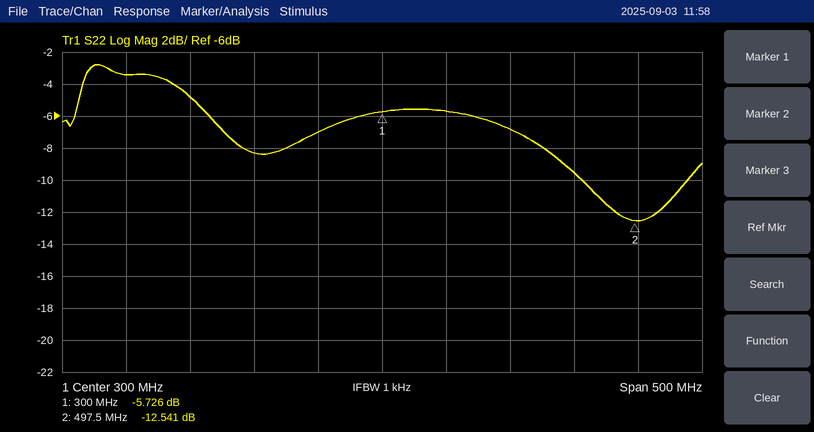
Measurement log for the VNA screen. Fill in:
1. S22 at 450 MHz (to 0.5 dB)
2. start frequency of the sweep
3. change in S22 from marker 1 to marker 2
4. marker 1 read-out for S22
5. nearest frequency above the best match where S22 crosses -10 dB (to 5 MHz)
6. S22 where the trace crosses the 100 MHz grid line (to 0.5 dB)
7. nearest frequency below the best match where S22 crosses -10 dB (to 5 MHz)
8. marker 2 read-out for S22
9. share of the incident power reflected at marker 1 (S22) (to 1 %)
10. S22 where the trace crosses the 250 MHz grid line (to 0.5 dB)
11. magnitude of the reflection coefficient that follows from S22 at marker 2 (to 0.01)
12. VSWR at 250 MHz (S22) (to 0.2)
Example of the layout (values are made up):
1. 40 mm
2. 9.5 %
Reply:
1. -9.5 dB
2. 50 MHz
3. -6.815 dB
4. -5.726 dB
5. 540 MHz
6. -3.5 dB
7. 455 MHz
8. -12.541 dB
9. 27 %
10. -7.0 dB
11. 0.24
12. 2.6
